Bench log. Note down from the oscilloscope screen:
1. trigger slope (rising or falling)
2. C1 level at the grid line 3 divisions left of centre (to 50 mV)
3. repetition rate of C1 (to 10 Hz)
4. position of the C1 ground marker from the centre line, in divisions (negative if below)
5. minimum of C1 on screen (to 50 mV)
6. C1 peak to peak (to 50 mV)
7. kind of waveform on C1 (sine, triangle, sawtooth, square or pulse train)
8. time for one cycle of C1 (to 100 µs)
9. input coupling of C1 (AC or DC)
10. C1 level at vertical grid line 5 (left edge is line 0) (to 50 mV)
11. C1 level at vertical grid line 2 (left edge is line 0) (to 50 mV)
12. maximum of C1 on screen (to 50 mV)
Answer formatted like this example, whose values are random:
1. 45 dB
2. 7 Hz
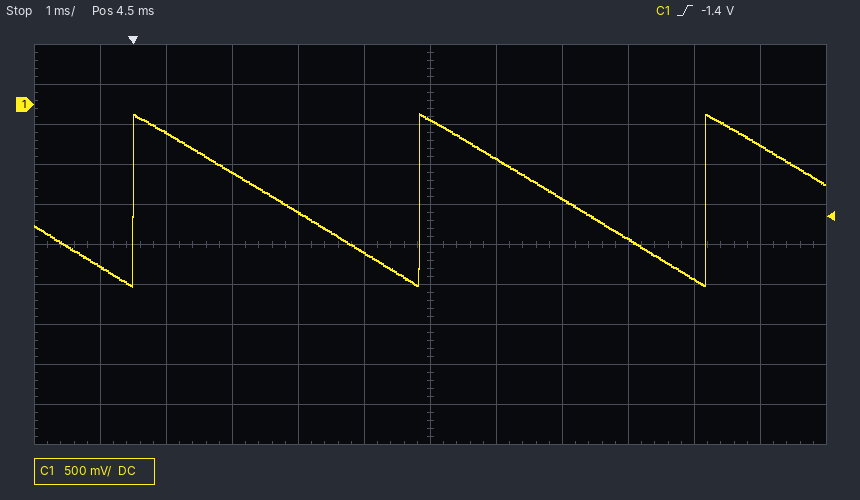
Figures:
1. rising
2. -850 mV
3. 230 Hz
4. +3.5 div
5. -2.25 V
6. 2.15 V
7. sawtooth
8. 4.3 ms
9. DC
10. -1.85 V
11. -350 mV
12. -100 mV
